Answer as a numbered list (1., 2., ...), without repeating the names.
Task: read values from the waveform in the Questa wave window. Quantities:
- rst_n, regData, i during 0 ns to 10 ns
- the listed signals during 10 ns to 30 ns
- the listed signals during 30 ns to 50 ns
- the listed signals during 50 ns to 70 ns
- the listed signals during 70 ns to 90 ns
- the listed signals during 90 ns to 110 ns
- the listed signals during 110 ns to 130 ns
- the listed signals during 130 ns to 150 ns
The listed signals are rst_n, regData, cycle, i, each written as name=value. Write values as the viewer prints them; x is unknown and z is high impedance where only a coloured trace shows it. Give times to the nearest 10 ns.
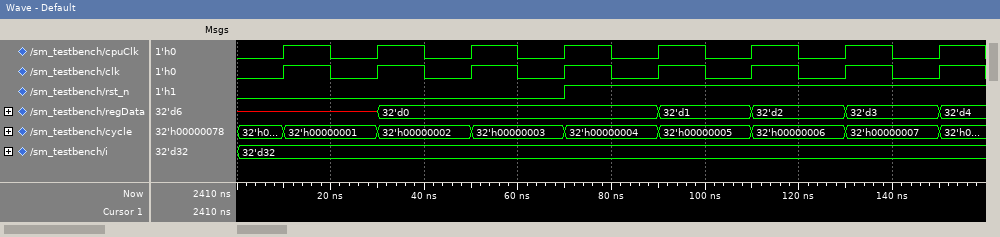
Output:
1. rst_n=0, regData=x, i=32'd32
2. rst_n=0, regData=x, cycle=32'h00000001, i=32'd32
3. rst_n=0, regData=32'd0, cycle=32'h00000002, i=32'd32
4. rst_n=0, regData=32'd0, cycle=32'h00000003, i=32'd32
5. rst_n=1, regData=32'd0, cycle=32'h00000004, i=32'd32
6. rst_n=1, regData=32'd1, cycle=32'h00000005, i=32'd32
7. rst_n=1, regData=32'd2, cycle=32'h00000006, i=32'd32
8. rst_n=1, regData=32'd3, cycle=32'h00000007, i=32'd32
